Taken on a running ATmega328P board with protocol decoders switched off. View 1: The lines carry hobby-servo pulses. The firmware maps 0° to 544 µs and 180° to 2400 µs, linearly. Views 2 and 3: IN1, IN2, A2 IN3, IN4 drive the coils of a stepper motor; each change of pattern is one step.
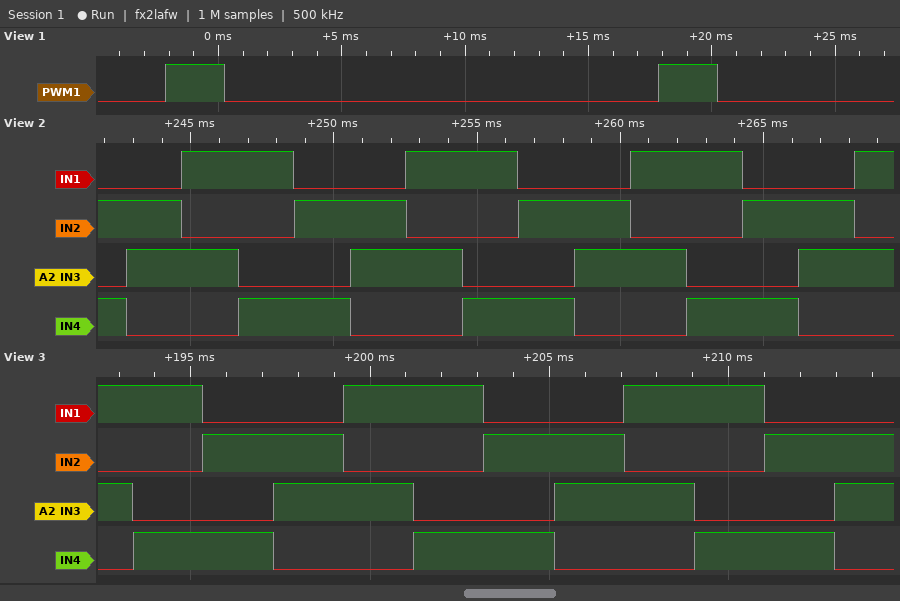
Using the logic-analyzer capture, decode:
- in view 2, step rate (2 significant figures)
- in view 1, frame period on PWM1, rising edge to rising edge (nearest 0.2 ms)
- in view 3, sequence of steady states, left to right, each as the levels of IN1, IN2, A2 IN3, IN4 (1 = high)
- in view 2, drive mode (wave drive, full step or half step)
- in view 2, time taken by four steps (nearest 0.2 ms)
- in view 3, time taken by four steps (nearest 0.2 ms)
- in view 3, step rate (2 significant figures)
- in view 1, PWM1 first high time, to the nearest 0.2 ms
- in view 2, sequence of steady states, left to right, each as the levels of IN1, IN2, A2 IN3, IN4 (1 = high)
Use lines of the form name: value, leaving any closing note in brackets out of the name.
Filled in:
in view 2, step rate: 510 steps/s
in view 1, frame period on PWM1, rising edge to rising edge: 20.0 ms
in view 3, sequence of steady states, left to right, each as the levels of IN1, IN2, A2 IN3, IN4: 1010 1001 0101 0110 1010 1001 0101 0110 1010 1001 0101 0110
in view 2, drive mode: full step
in view 2, time taken by four steps: 7.8 ms
in view 3, time taken by four steps: 7.8 ms
in view 3, step rate: 510 steps/s
in view 1, PWM1 first high time, to the nearest 0.2 ms: 2.4 ms
in view 2, sequence of steady states, left to right, each as the levels of IN1, IN2, A2 IN3, IN4: 0101 0110 1010 1001 0101 0110 1010 1001 0101 0110 1010 1001 0101 0110 1010
